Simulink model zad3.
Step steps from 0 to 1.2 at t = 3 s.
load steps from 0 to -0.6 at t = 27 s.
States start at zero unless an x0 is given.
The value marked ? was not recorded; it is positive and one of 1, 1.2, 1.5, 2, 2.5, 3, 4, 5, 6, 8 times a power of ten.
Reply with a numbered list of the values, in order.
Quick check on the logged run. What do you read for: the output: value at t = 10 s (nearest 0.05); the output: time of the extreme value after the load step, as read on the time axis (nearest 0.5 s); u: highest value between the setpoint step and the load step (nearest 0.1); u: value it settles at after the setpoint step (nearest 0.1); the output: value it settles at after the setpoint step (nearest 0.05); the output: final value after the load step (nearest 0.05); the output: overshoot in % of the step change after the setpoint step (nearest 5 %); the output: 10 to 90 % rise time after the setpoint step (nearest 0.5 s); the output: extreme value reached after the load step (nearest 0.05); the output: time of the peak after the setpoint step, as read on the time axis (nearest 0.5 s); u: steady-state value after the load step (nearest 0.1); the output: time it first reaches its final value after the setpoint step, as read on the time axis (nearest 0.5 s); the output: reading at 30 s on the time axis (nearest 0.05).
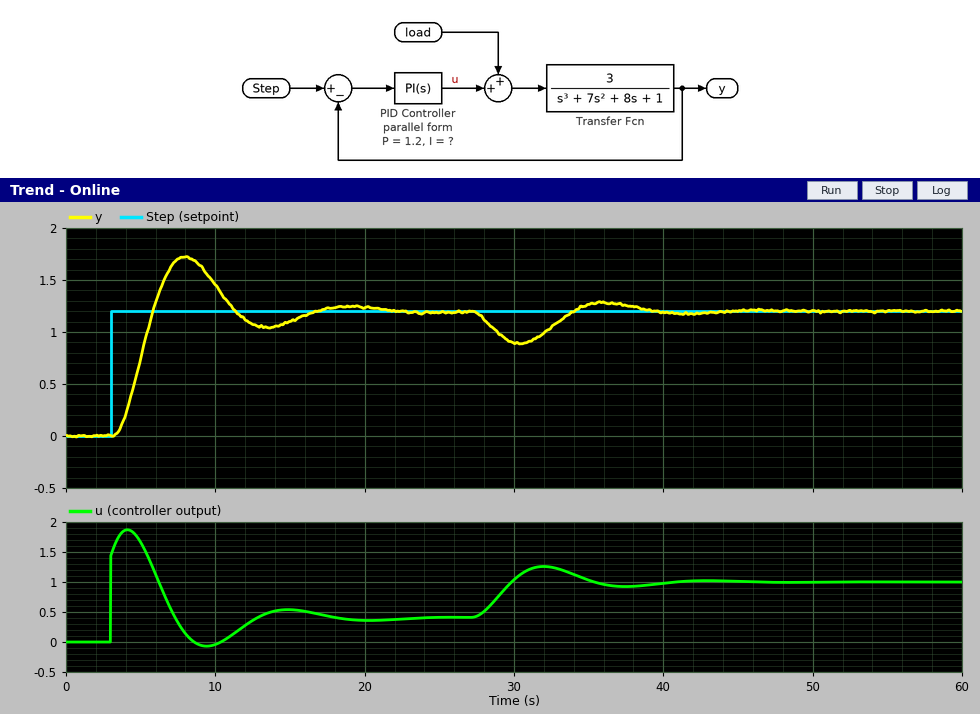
1. 1.45
2. 30.5 s
3. 1.9
4. 0.4
5. 1.20
6. 1.20
7. 45 %
8. 2.0 s
9. 0.90
10. 8.0 s
11. 1.0
12. 6.0 s
13. 0.90
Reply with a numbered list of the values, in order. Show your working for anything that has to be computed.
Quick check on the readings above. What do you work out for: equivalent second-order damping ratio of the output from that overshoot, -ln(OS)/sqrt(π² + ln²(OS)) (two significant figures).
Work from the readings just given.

1. ln(0.45) = -0.799; 0.799 / sqrt(9.870 + 0.638) = 0.25
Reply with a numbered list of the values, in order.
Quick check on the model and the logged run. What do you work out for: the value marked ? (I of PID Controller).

1. 0.6
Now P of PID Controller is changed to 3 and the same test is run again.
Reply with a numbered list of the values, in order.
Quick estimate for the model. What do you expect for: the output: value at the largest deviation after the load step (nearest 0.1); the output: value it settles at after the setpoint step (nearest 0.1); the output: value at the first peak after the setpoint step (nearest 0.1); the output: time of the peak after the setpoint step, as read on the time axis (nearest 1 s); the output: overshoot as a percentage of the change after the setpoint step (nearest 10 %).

1. 1.0
2. 1.2
3. 1.6
4. 6 s
5. 30 %
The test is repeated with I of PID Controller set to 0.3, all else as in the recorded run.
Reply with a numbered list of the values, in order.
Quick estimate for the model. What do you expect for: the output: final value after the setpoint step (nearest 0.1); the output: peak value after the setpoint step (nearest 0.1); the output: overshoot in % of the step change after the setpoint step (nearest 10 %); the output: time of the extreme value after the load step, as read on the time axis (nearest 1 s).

1. 1.2
2. 1.4
3. 20 %
4. 31 s
